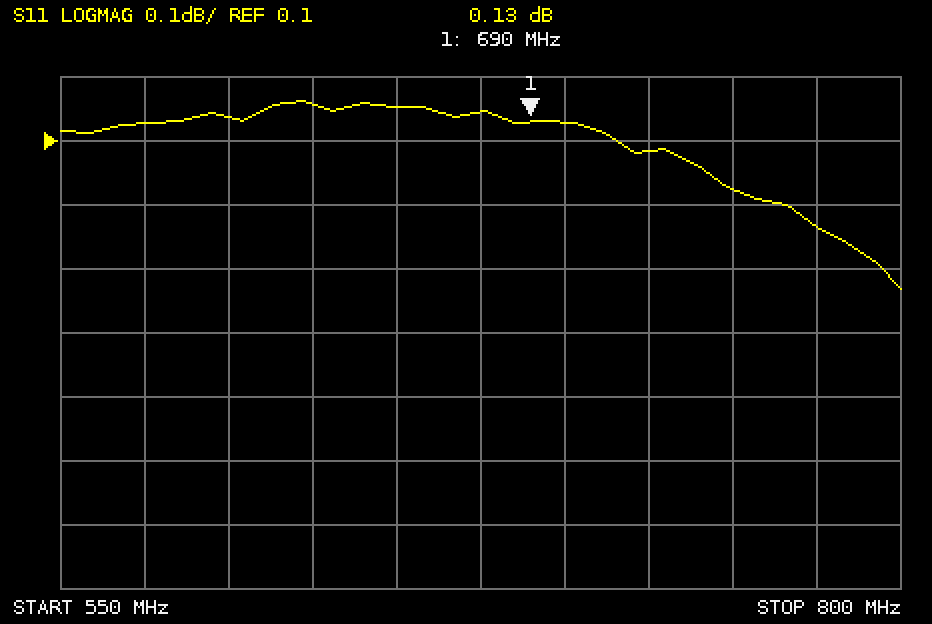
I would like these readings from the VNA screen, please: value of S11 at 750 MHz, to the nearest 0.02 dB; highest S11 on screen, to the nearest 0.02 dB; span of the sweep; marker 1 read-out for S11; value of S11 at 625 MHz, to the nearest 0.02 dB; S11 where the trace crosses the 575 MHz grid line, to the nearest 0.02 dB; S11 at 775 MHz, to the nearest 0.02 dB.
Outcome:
0.02 dB
0.16 dB
250 MHz
0.13 dB
0.16 dB
0.12 dB
-0.04 dB
